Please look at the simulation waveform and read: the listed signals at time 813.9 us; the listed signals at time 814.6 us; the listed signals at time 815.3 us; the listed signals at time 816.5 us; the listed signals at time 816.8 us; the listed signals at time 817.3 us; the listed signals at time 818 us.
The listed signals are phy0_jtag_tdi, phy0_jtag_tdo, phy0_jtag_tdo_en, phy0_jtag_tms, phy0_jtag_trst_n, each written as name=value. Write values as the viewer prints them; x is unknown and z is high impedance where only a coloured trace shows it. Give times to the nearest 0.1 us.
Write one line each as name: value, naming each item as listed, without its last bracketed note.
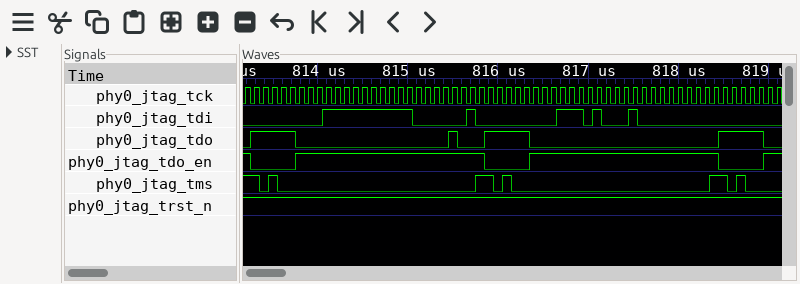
the listed signals at time 813.9 us: phy0_jtag_tdi=0, phy0_jtag_tdo=0, phy0_jtag_tdo_en=1, phy0_jtag_tms=0, phy0_jtag_trst_n=1
the listed signals at time 814.6 us: phy0_jtag_tdi=1, phy0_jtag_tdo=0, phy0_jtag_tdo_en=1, phy0_jtag_tms=0, phy0_jtag_trst_n=1
the listed signals at time 815.3 us: phy0_jtag_tdi=0, phy0_jtag_tdo=0, phy0_jtag_tdo_en=1, phy0_jtag_tms=0, phy0_jtag_trst_n=1
the listed signals at time 816.5 us: phy0_jtag_tdi=0, phy0_jtag_tdo=0, phy0_jtag_tdo_en=1, phy0_jtag_tms=0, phy0_jtag_trst_n=1
the listed signals at time 816.8 us: phy0_jtag_tdi=1, phy0_jtag_tdo=0, phy0_jtag_tdo_en=1, phy0_jtag_tms=0, phy0_jtag_trst_n=1
the listed signals at time 817.3 us: phy0_jtag_tdi=0, phy0_jtag_tdo=0, phy0_jtag_tdo_en=1, phy0_jtag_tms=0, phy0_jtag_trst_n=1
the listed signals at time 818 us: phy0_jtag_tdi=0, phy0_jtag_tdo=0, phy0_jtag_tdo_en=1, phy0_jtag_tms=0, phy0_jtag_trst_n=1
